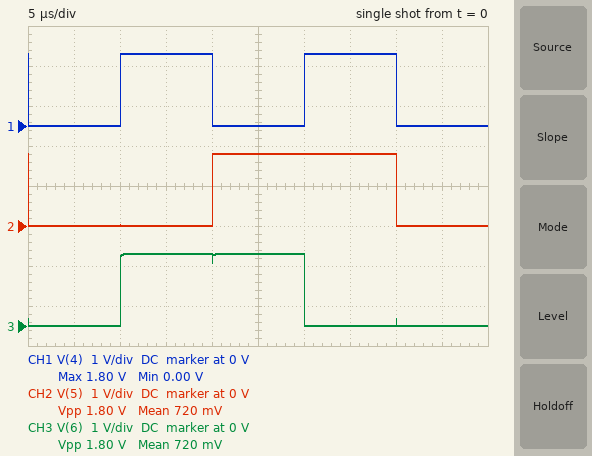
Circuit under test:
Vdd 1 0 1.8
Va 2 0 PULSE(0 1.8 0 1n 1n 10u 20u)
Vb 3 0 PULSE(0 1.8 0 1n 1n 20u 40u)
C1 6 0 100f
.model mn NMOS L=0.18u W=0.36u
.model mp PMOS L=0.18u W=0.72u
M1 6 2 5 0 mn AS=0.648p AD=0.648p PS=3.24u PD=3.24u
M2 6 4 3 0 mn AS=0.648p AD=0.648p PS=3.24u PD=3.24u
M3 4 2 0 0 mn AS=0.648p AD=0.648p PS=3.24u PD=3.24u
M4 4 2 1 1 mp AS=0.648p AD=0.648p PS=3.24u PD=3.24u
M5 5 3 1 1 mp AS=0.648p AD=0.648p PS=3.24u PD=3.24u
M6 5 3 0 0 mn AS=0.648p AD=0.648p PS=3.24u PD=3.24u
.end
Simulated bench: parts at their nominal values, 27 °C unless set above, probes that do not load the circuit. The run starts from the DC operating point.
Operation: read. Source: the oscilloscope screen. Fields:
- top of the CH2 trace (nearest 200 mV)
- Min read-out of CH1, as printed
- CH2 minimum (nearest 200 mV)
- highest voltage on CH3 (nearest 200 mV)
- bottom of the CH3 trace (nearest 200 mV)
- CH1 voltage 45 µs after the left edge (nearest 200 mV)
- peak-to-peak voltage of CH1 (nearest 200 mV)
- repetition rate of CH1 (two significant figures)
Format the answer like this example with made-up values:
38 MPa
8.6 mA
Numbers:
1.8 V
0.00 V
0 V
1.8 V
0 V
0 V
1.8 V
50 kHz
